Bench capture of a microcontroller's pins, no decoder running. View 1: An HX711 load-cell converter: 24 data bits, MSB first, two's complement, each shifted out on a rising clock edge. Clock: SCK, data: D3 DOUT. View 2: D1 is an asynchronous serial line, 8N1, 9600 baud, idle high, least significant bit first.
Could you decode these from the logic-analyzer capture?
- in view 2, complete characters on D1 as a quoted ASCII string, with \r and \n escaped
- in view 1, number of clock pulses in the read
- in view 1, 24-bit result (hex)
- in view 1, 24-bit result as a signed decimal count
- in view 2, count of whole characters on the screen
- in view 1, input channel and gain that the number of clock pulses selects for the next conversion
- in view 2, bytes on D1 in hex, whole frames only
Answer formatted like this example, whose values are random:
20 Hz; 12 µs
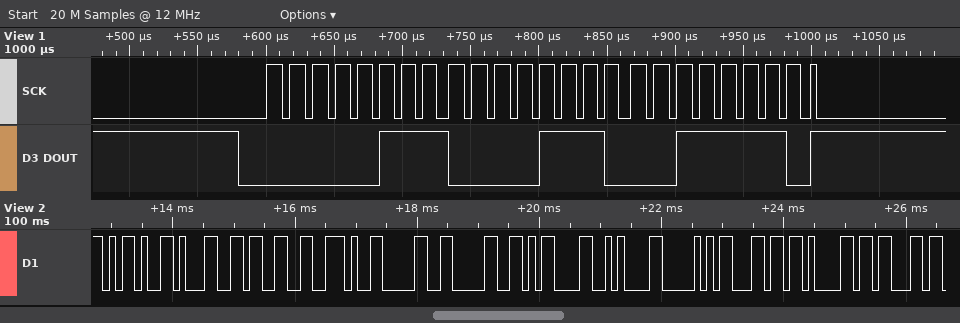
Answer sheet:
"-13.00\r\nPlac"; 25; 0x070E3E; 462398; 12; channel A, gain 128; 2D 31 33 2E 30 30 0D 0A 50 6C 61 63
